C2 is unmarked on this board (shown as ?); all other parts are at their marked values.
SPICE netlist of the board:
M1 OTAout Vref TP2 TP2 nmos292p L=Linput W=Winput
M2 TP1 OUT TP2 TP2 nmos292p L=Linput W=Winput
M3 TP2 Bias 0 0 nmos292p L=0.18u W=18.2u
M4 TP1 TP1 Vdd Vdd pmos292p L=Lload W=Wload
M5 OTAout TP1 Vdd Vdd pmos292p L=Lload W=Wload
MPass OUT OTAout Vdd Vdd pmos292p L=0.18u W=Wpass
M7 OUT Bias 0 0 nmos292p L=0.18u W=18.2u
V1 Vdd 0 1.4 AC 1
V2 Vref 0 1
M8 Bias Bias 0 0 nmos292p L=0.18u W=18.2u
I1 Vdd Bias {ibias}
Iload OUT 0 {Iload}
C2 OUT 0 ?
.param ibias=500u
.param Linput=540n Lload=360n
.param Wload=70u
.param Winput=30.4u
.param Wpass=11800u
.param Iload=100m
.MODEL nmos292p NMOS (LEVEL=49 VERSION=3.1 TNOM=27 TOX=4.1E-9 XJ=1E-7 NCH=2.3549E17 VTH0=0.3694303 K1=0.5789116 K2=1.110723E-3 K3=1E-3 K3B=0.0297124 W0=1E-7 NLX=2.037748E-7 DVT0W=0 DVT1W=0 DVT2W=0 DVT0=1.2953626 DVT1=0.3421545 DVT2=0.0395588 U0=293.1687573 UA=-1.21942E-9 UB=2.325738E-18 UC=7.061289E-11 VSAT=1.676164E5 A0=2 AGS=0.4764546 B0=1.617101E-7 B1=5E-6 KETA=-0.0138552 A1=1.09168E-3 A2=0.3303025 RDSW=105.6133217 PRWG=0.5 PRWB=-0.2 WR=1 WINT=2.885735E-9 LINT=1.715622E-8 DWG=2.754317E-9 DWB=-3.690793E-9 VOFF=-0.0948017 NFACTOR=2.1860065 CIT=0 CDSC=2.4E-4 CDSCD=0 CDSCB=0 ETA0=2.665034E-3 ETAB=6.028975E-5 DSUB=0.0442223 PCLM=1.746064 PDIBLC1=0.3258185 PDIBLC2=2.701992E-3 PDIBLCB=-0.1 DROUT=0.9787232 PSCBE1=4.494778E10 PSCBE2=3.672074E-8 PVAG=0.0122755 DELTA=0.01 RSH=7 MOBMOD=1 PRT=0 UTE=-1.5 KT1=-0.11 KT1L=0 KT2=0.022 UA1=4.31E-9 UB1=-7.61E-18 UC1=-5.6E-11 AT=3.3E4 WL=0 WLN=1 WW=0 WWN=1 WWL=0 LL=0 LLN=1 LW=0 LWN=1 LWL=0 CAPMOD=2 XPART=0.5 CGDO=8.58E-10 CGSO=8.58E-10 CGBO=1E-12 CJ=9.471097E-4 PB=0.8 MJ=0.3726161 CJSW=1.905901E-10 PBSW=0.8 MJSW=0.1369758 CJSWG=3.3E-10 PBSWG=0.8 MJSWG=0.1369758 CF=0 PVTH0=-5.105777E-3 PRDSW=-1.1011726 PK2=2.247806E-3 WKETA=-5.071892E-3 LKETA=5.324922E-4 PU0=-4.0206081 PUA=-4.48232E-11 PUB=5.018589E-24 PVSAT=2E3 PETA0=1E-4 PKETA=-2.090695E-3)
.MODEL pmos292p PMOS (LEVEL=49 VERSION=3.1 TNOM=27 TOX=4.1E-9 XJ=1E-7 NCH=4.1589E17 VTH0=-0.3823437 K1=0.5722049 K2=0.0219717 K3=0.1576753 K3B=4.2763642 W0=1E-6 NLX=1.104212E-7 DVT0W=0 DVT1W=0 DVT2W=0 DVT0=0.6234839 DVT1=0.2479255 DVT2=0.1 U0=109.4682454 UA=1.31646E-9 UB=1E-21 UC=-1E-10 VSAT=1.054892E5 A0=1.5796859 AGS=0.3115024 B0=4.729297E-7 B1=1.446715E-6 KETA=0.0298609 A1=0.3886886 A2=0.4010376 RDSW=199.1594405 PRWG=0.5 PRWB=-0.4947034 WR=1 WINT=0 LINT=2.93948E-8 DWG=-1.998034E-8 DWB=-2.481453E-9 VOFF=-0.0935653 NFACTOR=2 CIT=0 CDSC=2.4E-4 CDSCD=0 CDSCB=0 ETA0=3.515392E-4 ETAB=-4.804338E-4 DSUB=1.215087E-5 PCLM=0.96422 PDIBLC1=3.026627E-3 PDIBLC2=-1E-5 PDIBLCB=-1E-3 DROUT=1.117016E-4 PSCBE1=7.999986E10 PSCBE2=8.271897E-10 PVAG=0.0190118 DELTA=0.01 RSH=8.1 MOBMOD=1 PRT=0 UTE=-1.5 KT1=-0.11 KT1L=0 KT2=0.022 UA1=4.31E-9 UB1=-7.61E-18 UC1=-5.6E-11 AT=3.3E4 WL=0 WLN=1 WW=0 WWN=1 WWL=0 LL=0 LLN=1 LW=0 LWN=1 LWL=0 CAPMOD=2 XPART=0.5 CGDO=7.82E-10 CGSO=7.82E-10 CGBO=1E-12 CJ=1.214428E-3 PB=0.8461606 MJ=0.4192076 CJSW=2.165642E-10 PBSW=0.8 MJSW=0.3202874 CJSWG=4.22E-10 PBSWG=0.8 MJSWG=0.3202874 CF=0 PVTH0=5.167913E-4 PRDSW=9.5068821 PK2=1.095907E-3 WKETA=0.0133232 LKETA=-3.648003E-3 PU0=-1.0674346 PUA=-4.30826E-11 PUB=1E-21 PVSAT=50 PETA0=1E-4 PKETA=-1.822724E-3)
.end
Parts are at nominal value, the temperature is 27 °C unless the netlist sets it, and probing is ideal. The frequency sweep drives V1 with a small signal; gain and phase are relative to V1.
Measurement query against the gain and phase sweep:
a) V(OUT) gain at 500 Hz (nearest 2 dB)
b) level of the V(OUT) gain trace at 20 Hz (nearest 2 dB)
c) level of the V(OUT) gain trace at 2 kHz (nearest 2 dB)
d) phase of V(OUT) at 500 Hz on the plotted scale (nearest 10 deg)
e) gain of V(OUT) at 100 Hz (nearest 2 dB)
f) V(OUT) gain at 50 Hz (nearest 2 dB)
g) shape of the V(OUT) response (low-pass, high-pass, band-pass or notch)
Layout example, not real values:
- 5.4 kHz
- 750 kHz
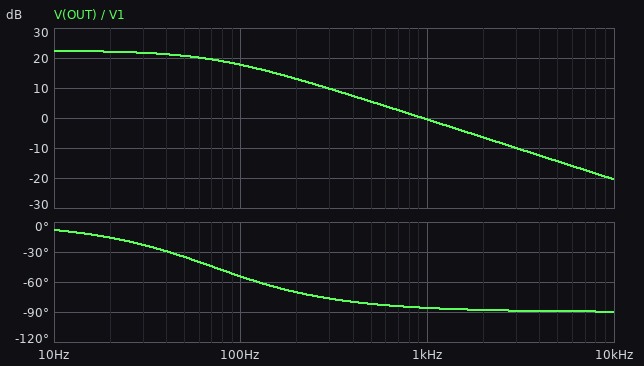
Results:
- 6 dB
- 22 dB
- -6 dB
- -80 deg
- 18 dB
- 20 dB
- low-pass
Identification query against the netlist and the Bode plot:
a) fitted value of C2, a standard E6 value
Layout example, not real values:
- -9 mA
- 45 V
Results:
- 15 µF
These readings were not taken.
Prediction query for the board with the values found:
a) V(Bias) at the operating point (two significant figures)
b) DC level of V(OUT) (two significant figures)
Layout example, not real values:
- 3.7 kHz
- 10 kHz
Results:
- 660 mV
- -3.1 V
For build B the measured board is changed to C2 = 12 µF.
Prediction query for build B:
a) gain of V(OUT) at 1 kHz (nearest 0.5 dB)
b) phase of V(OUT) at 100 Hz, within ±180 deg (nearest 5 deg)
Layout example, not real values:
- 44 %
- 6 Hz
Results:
- 1.5 dB
- -50 deg
